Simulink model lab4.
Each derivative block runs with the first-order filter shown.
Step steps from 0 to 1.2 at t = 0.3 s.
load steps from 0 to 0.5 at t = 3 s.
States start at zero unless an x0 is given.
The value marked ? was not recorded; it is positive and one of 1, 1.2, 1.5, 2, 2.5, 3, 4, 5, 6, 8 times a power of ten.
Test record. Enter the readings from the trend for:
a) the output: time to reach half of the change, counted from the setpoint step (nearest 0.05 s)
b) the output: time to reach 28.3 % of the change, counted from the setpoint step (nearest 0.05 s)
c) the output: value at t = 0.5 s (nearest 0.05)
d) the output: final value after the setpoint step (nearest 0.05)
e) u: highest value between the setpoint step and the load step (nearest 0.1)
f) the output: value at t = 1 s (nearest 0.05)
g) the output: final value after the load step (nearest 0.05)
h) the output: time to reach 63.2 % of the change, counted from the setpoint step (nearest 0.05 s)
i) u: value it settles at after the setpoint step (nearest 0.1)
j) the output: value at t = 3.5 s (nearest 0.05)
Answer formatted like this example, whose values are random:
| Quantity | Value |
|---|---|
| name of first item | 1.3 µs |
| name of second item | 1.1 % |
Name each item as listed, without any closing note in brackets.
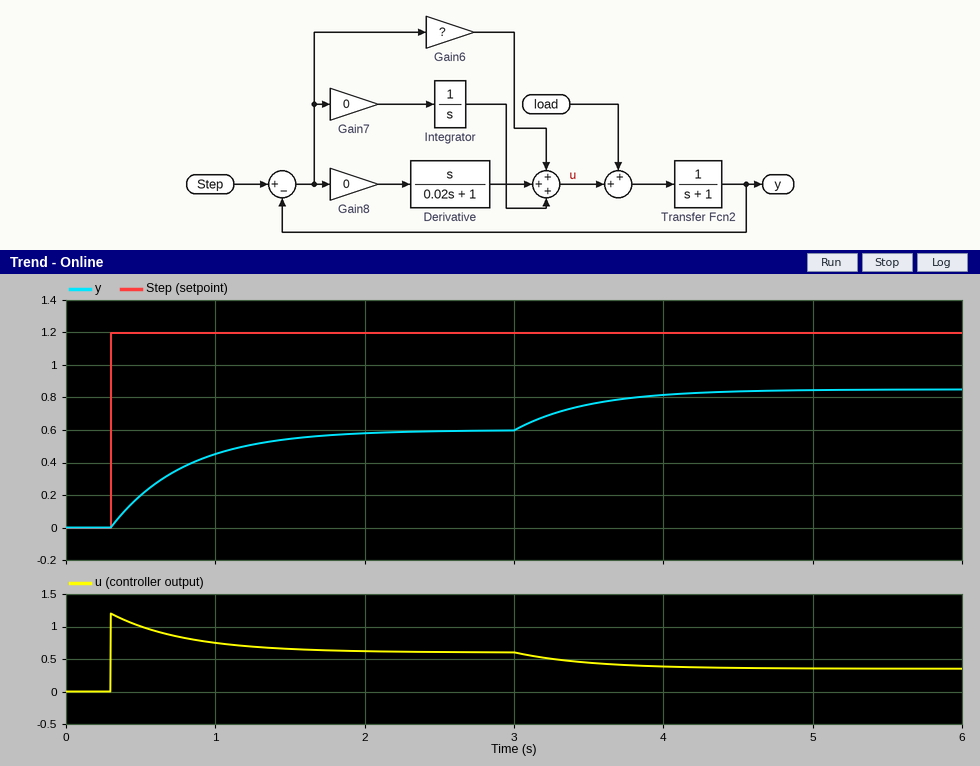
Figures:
| Quantity | Value |
|---|---|
| the output: time to reach half of the change, counted from the setpoint step | 0.35 s |
| the output: time to reach 28.3 % of the change, counted from the setpoint step | 0.15 s |
| the output: value at t = 0.5 s | 0.20 |
| the output: final value after the setpoint step | 0.60 |
| u: highest value between the setpoint step and the load step | 1.2 |
| the output: value at t = 1 s | 0.45 |
| the output: final value after the load step | 0.85 |
| the output: time to reach 63.2 % of the change, counted from the setpoint step | 0.50 s |
| u: value it settles at after the setpoint step | 0.6 |
| the output: value at t = 3.5 s | 0.75 |
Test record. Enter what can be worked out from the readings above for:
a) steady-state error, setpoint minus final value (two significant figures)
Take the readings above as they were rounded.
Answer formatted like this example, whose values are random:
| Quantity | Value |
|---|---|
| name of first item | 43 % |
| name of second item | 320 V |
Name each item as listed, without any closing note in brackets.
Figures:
| Quantity | Value |
|---|---|
| steady-state error, setpoint minus final value | 0.60 |
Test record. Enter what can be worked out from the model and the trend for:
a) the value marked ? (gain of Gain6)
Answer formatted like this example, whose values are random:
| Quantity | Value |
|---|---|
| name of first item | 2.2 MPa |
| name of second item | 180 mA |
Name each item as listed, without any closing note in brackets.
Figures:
| Quantity | Value |
|---|---|
| the value marked ? | 1 |
